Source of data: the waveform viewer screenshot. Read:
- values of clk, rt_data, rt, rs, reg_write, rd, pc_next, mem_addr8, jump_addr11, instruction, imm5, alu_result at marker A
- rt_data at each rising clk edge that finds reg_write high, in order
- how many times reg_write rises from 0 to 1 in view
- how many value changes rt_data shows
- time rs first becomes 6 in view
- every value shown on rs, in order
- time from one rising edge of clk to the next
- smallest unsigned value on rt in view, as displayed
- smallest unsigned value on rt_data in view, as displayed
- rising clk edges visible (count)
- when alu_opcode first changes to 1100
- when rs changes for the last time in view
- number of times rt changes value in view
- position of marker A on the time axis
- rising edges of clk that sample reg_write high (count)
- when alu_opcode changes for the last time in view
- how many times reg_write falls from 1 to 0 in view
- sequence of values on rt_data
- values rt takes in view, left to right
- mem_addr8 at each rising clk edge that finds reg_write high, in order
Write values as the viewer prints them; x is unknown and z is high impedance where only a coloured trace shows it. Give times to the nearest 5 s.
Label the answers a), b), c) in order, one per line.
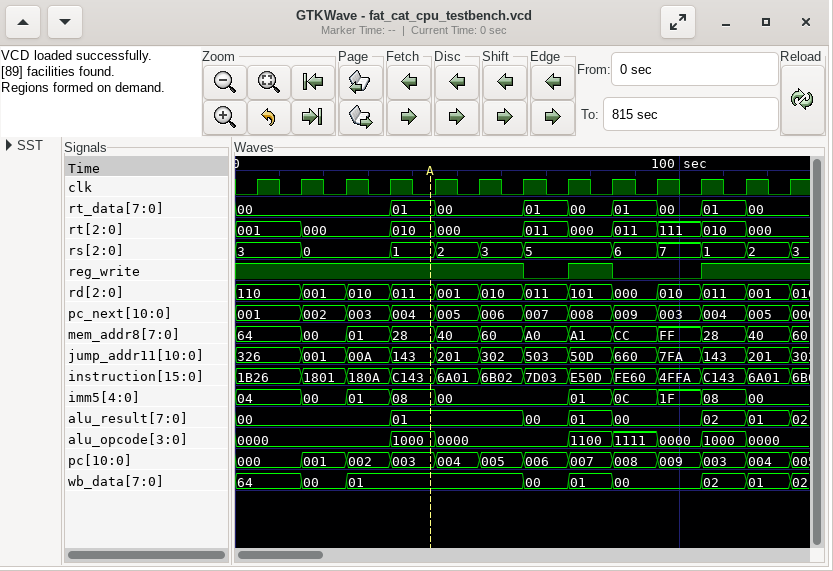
a) clk=0, rt_data=01, rt=010, rs=1, reg_write=1, rd=011, pc_next=004, mem_addr8=28, jump_addr11=143, instruction=C143, imm5=08, alu_result=01
b) 00, 00, 00, 00, 01, 00, 00, 00, 01, 00
c) 2
d) 8
e) 85 s
f) 3, 0, 1, 2, 3, 5, 6, 7, 1, 2, 3
g) 10 s
h) 000
i) 00
j) 13
k) 75 s
l) 125 s
m) 9
n) 45 s
o) 10
p) 115 s
q) 2
r) 00, 01, 00, 01, 00, 01, 00, 01, 00
s) 001, 000, 010, 000, 011, 000, 011, 111, 010, 000
t) 64, 64, 00, 01, 28, 40, 60, A1, 28, 40
